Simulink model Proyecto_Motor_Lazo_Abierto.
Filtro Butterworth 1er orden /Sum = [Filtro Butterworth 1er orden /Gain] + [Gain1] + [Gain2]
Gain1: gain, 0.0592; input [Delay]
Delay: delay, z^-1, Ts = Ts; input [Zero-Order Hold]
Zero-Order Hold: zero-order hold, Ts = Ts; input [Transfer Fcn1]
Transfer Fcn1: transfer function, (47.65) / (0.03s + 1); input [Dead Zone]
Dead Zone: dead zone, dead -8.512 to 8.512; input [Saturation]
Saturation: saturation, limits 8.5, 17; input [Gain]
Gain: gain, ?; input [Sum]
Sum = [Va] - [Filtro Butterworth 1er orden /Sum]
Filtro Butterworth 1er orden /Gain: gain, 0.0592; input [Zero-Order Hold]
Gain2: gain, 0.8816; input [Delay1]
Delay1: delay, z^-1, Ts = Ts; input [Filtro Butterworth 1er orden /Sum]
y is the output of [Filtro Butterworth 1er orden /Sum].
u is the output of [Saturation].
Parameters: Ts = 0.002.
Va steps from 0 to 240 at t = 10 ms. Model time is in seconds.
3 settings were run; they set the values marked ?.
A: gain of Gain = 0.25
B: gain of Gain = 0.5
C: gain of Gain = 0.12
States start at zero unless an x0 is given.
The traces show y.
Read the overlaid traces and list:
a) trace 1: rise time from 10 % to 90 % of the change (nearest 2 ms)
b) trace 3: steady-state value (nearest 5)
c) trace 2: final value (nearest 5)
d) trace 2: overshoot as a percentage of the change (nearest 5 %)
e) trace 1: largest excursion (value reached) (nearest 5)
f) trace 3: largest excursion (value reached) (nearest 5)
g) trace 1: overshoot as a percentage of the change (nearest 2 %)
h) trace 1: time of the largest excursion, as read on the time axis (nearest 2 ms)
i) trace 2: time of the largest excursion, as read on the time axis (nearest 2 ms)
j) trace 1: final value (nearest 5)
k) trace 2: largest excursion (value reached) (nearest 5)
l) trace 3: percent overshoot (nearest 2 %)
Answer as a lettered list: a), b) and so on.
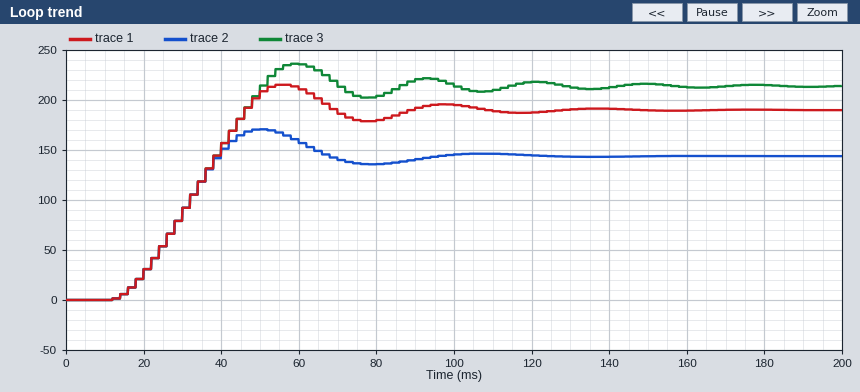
a) 26 ms
b) 215
c) 145
d) 20 %
e) 215
f) 235
g) 14 %
h) 56 ms
i) 50 ms
j) 190
k) 170
l) 10 %
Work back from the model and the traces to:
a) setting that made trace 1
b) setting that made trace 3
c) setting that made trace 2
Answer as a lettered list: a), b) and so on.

a) A
b) B
c) C
